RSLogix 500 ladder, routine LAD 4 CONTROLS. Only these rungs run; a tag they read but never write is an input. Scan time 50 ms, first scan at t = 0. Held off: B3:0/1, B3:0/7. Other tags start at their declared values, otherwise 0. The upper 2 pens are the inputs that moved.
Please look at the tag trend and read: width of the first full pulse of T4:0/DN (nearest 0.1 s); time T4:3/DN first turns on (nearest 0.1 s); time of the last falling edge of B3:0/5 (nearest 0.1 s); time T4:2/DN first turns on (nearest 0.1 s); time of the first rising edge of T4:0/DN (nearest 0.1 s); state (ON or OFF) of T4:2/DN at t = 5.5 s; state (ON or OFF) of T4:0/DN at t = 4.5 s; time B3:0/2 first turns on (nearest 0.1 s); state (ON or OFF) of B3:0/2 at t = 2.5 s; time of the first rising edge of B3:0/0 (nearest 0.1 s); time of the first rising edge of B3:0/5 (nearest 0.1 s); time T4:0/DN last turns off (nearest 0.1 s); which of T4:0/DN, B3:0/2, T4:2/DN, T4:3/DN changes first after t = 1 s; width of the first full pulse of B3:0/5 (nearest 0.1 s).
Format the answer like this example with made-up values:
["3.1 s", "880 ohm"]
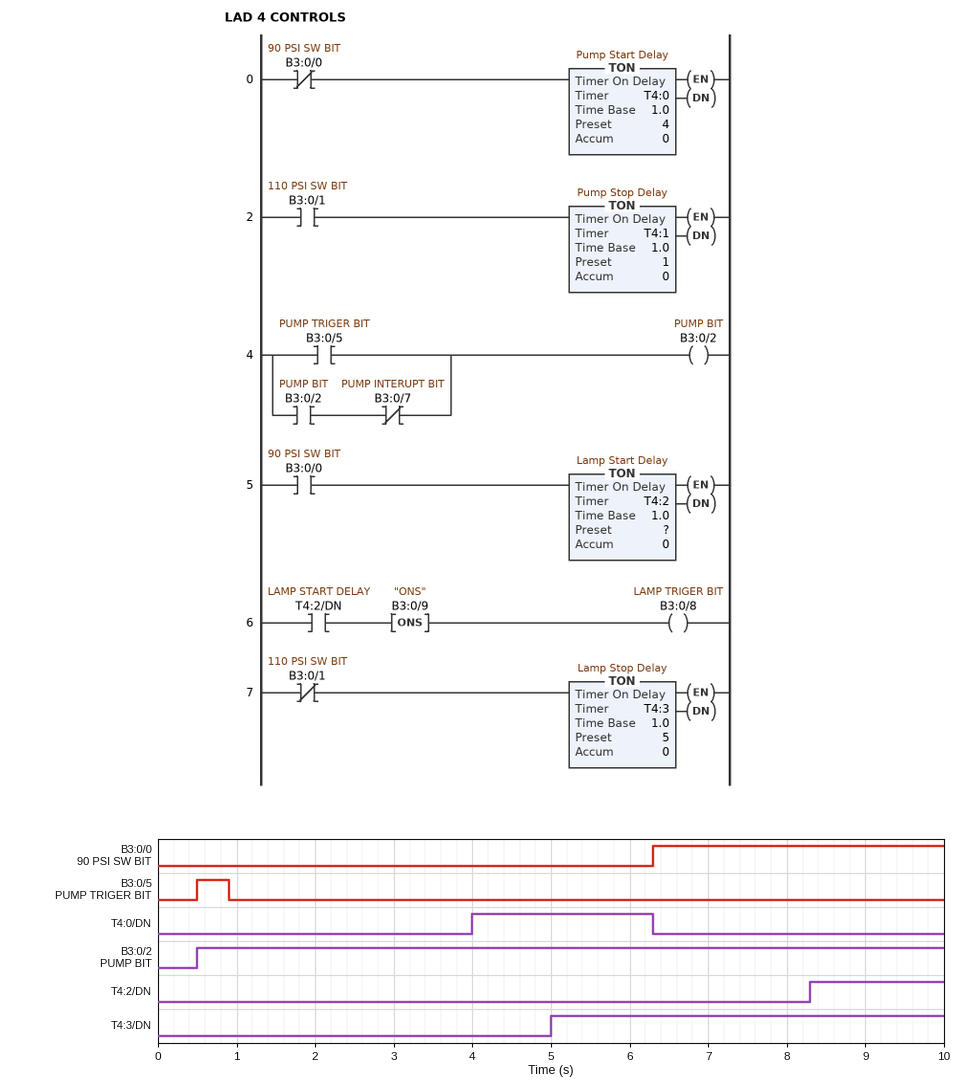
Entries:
["2.3 s", "5.0 s", "0.9 s", "8.3 s", "4.0 s", "OFF", "ON", "0.5 s", "ON", "6.3 s", "0.5 s", "6.3 s", "T4:0/DN", "0.4 s"]
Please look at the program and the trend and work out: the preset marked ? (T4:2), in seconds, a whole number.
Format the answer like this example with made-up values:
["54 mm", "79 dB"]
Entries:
["2 s"]
